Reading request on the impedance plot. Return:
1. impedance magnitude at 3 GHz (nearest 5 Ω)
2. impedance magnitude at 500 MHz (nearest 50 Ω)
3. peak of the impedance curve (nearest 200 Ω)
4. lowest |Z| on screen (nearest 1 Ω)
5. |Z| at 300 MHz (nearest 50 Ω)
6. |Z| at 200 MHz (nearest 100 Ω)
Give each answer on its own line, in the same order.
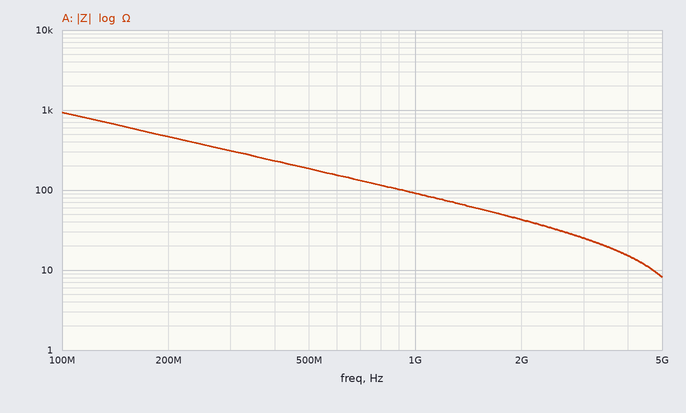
25 Ω
200 Ω
1.0 kΩ
8 Ω
300 Ω
500 Ω
